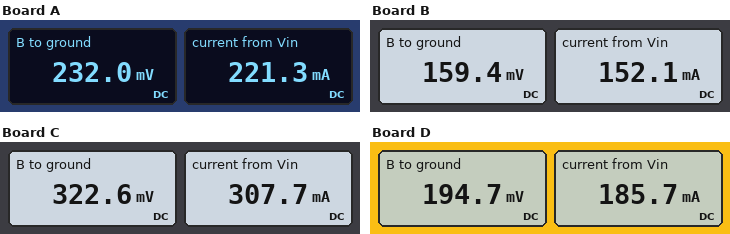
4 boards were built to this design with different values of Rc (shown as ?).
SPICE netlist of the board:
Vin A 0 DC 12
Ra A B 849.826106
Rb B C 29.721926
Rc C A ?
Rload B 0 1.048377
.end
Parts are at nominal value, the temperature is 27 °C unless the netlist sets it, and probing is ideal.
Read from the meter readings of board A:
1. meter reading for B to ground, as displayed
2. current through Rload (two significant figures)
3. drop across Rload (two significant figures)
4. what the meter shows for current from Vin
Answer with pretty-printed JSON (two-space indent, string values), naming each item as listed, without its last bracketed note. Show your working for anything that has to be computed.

{
  "meter reading for B to ground, as displayed": "232.0 mV",
  "current through Rload": "(232 mV) / 1.048 Ω = 220 mA",
  "drop across Rload": "232 mV = 230 mV",
  "what the meter shows for current from Vin": "221.3 mA"
}
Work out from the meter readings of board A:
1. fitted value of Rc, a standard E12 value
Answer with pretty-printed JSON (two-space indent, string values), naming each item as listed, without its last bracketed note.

{
  "fitted value of Rc, a standard E12 value": "27 Ω"
}
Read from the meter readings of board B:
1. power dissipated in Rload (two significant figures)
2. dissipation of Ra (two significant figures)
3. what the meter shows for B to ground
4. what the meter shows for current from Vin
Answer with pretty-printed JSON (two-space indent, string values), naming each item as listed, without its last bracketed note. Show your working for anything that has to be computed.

{
  "power dissipated in Rload": "(159.4 mV)^2 / 1.048 Ω = 24 mW",
  "dissipation of Ra": "(12 V - 159.4 mV)^2 / 849.8 Ω = 160 mW",
  "what the meter shows for B to ground": "159.4 mV",
  "what the meter shows for current from Vin": "152.1 mA"
}
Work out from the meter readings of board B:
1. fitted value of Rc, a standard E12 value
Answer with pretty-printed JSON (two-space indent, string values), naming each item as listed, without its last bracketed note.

{
  "fitted value of Rc, a standard E12 value": "56 Ω"
}
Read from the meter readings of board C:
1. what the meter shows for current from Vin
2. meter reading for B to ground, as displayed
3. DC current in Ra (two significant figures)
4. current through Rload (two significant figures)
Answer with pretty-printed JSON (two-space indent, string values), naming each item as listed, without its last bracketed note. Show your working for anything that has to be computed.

{
  "what the meter shows for current from Vin": "307.7 mA",
  "meter reading for B to ground, as displayed": "322.6 mV",
  "DC current in Ra": "(12 V - 322.6 mV) / 849.8 Ω = 14 mA",
  "current through Rload": "(322.6 mV) / 1.048 Ω = 310 mA"
}
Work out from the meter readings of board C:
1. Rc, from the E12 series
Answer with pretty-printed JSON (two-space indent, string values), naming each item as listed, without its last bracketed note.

{
  "Rc, from the E12 series": "10 Ω"
}
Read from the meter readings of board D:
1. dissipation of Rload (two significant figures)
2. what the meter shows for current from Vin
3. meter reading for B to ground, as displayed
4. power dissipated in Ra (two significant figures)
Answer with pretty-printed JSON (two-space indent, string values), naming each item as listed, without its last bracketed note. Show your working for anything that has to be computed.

{
  "dissipation of Rload": "(194.7 mV)^2 / 1.048 Ω = 36 mW",
  "what the meter shows for current from Vin": "185.7 mA",
  "meter reading for B to ground, as displayed": "194.7 mV",
  "power dissipated in Ra": "(12 V - 194.7 mV)^2 / 849.8 Ω = 160 mW"
}
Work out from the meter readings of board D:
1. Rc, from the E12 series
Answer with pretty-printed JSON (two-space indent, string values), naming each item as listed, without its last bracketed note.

{
  "Rc, from the E12 series": "39 Ω"
}
